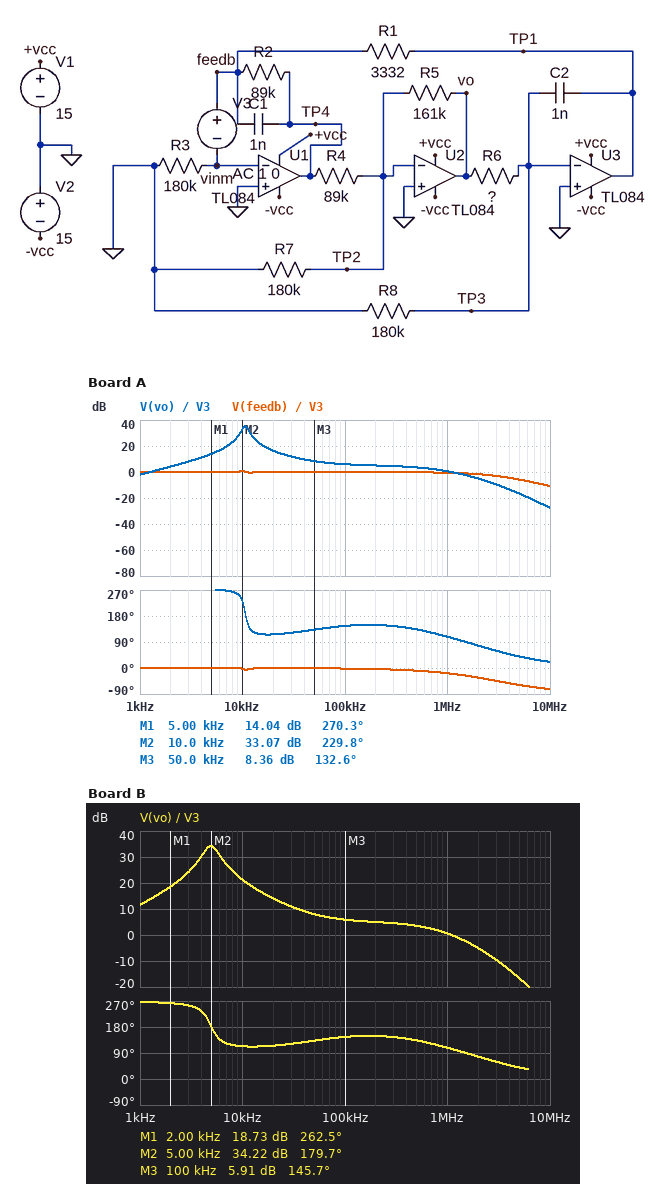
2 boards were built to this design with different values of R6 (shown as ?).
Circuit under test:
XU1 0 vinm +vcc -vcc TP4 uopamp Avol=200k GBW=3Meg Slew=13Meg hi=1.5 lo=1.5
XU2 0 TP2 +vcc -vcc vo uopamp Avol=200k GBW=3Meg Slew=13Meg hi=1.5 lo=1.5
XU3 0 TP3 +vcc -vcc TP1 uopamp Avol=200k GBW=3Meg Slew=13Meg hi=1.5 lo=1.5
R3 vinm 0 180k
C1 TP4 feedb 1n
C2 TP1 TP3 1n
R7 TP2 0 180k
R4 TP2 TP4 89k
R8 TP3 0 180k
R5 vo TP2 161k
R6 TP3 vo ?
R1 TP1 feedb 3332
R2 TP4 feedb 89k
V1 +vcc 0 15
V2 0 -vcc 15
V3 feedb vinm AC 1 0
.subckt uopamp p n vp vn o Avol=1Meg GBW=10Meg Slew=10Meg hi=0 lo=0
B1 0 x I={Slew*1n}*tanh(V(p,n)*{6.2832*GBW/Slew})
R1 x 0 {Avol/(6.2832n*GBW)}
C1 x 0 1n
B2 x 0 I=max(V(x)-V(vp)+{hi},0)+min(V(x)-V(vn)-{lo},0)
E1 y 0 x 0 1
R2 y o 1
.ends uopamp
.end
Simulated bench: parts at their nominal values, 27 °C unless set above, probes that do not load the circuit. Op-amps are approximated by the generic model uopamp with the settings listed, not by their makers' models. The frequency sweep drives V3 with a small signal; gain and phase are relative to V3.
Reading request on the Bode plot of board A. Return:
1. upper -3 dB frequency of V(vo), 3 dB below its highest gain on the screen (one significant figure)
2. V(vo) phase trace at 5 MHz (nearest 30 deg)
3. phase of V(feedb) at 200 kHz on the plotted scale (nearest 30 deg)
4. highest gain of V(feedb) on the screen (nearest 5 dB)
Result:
10 kHz
30 deg
0 deg
0 dB
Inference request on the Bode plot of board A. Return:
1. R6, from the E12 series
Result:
120 kΩ
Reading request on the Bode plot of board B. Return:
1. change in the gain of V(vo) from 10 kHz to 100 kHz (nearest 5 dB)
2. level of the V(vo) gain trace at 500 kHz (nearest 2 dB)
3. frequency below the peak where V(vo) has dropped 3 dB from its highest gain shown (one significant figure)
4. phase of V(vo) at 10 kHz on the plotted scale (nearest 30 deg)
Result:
-15 dB
4 dB
4 kHz
120 deg
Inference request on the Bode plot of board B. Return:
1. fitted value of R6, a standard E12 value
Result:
560 kΩ
